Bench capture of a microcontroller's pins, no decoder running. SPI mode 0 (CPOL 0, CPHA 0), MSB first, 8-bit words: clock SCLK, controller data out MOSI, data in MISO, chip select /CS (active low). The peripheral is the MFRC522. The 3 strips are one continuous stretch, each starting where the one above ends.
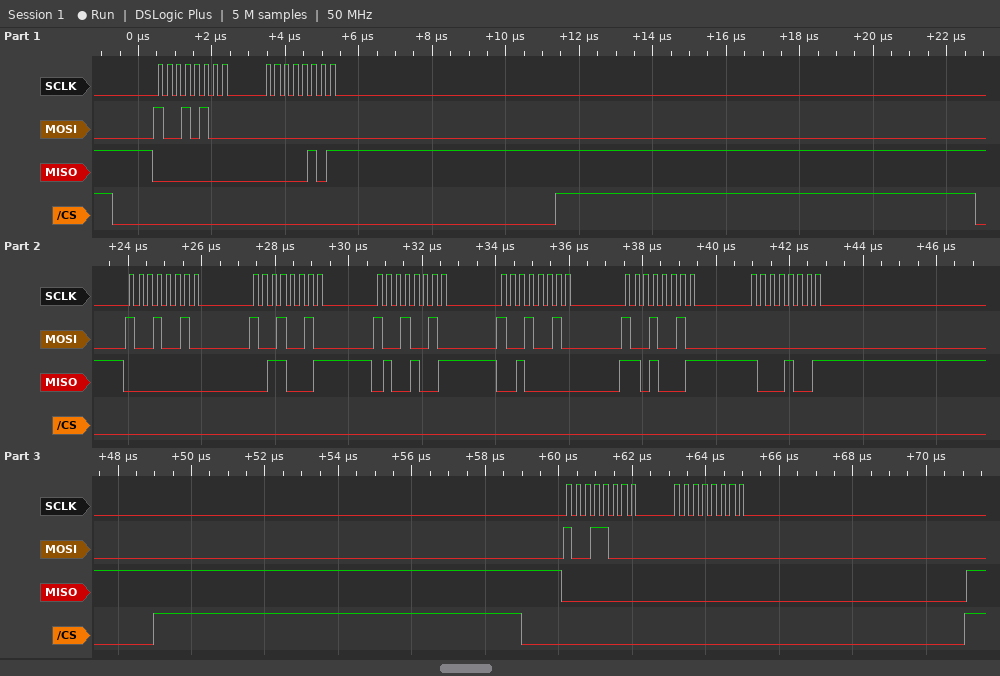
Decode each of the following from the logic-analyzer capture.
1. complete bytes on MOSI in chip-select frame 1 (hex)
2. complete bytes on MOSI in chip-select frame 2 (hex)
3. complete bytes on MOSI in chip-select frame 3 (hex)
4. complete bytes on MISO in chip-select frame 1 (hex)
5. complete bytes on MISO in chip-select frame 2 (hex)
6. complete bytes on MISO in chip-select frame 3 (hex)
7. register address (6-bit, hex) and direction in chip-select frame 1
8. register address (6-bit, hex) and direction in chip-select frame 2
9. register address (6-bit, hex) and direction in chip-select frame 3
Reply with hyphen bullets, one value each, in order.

- 94 00
- 92 92 92 92 92 00
- 98 00
- 00 05
- 00 31 49 20 D1 89
- 00 00
- 0x0A read
- 0x09 read
- 0x0C read
